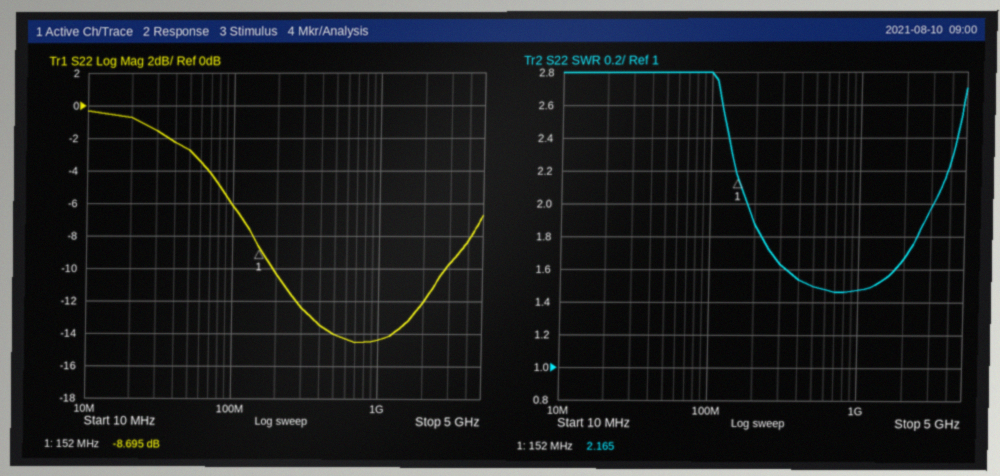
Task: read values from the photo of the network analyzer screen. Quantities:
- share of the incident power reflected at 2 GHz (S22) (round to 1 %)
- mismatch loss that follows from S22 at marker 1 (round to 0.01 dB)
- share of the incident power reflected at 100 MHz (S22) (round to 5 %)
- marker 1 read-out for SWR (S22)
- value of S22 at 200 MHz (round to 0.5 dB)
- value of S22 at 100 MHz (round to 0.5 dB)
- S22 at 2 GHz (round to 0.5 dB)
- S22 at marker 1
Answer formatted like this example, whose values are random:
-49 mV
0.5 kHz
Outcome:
6 %
0.63 dB
25 %
2.165
-10.5 dB
-6.0 dB
-12.0 dB
-8.695 dB
